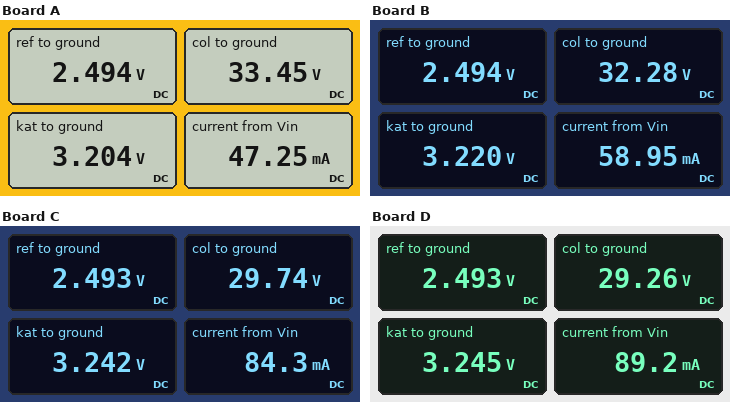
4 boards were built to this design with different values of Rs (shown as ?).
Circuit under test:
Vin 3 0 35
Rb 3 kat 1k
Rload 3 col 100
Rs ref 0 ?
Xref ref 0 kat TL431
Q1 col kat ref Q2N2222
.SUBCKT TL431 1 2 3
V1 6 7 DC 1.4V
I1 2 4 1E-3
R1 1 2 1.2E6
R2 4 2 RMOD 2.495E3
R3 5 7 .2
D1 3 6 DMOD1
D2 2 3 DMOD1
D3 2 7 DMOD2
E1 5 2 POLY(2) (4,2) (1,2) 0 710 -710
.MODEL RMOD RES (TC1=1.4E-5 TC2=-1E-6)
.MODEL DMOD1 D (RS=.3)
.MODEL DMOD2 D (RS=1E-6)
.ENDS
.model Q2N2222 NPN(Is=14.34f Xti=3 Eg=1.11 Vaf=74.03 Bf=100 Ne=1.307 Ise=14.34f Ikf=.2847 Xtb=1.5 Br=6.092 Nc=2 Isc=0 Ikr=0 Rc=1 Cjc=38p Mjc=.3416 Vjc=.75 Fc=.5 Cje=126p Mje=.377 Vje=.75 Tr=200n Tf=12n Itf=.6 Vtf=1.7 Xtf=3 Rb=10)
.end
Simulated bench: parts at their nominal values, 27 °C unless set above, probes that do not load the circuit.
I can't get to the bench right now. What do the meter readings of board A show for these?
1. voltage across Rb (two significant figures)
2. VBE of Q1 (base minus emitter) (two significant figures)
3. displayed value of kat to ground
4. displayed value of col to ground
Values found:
32 V
710 mV
3.204 V
33.45 V
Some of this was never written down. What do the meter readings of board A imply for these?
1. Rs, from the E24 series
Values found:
160 Ω
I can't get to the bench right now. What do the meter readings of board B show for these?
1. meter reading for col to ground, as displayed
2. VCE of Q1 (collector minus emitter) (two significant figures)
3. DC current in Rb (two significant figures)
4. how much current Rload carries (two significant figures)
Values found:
32.28 V
30 V
32 mA
27 mA
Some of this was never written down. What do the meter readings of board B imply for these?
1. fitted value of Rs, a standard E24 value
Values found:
91 Ω
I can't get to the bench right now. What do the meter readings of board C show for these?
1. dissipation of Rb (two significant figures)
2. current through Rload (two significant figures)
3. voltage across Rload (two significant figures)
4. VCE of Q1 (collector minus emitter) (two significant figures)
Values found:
1.0 W
53 mA
5.3 V
27 V
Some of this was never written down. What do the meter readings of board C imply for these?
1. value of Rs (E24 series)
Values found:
47 Ω
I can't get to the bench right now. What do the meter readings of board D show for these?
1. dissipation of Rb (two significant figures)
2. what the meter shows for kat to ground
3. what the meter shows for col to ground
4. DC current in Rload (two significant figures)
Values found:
1.0 W
3.245 V
29.26 V
57 mA
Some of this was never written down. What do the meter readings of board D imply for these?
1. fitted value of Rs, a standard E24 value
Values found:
43 Ω
